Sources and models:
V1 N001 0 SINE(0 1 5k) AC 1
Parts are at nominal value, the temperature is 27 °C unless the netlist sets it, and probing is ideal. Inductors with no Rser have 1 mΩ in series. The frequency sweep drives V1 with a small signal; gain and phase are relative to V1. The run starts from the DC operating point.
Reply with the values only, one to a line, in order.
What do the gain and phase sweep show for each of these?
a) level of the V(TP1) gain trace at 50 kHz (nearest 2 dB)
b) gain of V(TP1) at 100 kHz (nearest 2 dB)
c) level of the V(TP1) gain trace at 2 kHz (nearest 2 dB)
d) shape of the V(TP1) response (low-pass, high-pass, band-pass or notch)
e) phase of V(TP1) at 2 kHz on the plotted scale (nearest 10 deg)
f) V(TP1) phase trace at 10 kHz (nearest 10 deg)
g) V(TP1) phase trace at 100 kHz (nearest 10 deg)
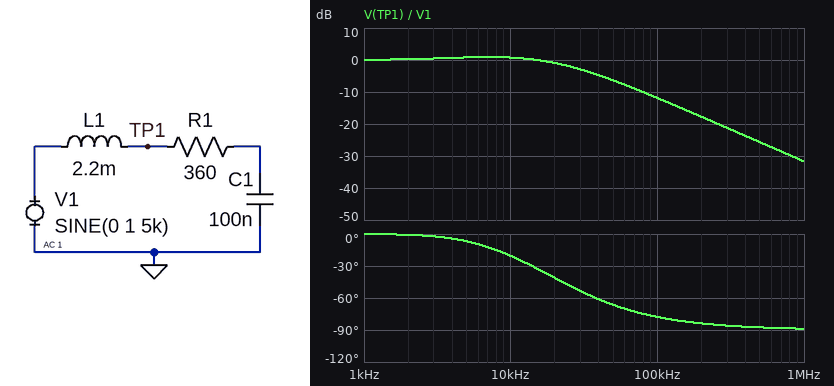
-6 dB
-12 dB
0 dB
low-pass
0 deg
-20 deg
-80 deg
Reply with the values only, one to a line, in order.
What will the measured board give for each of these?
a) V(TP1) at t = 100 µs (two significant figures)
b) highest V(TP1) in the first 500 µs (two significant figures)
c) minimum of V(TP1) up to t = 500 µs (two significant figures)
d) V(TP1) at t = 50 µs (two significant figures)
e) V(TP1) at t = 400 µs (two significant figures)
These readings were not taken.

120 mV
1.1 V
-1.1 V
1.1 V
-130 mV
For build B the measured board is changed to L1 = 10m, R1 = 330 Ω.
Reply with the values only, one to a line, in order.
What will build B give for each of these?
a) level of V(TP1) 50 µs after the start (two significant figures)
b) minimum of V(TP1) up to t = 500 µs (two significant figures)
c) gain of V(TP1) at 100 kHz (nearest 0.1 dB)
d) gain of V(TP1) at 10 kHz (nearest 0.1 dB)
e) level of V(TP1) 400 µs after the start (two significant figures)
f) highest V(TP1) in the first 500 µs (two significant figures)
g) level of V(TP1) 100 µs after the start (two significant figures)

850 mV
-1.4 V
-25.6 dB
-3.9 dB
-950 mV
1.4 V
740 mV
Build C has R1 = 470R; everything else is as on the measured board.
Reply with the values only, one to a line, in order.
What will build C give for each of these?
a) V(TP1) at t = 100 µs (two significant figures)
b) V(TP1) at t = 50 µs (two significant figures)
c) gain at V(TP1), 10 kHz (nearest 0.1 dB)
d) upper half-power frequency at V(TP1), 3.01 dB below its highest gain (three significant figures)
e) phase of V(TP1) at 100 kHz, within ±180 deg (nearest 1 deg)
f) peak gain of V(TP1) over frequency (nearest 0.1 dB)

110 mV
1.0 V
0.5 dB
33.2 kHz
-73 deg
0.6 dB
